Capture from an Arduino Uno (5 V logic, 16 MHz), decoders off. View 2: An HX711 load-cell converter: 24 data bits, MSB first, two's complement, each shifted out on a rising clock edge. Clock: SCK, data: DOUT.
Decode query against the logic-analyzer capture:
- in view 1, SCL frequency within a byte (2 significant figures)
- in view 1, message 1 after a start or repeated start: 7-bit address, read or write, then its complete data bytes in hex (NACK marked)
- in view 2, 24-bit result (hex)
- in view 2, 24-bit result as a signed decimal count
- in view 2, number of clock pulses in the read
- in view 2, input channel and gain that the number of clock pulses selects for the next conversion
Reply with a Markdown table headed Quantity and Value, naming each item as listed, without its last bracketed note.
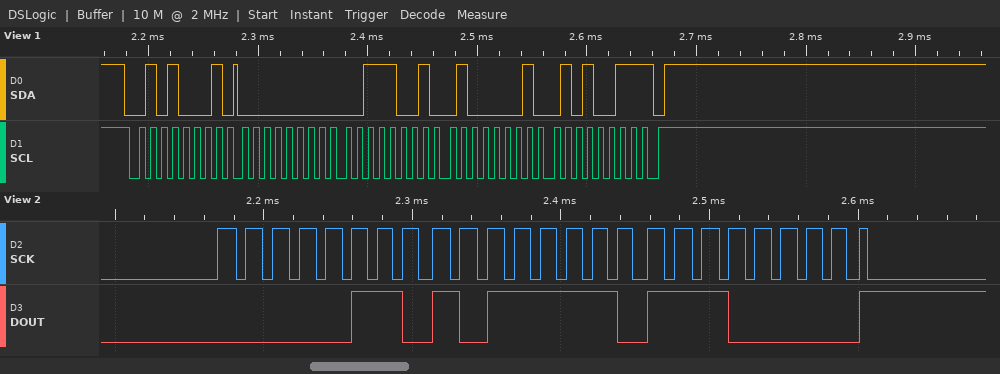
| Quantity | Value |
|---|---|
| in view 1, SCL frequency within a byte | 100 kHz |
| in view 1, message 1 after a start or repeated start: 7-bit address, read or write, then its complete data bytes in hex | 0x28 read: 00 39 41 53 NACK |
| in view 2, 24-bit result | 0x06BEE0 |
| in view 2, 24-bit result as a signed decimal count | 442080 |
| in view 2, number of clock pulses in the read | 25 |
| in view 2, input channel and gain that the number of clock pulses selects for the next conversion | channel A, gain 128 |
